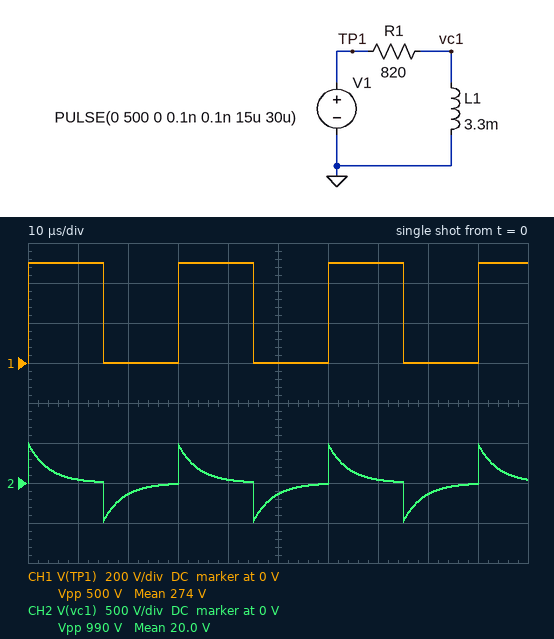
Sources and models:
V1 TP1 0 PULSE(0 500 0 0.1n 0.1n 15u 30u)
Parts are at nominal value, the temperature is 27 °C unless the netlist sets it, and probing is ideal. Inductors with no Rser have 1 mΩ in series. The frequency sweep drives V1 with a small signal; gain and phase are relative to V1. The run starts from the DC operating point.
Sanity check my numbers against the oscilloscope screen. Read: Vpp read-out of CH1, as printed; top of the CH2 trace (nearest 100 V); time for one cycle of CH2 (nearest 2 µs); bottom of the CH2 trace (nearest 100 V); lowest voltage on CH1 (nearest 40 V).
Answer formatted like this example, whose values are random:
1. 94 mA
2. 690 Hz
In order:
1. 500 V
2. 500 V
3. 30 µs
4. -500 V
5. 0 V
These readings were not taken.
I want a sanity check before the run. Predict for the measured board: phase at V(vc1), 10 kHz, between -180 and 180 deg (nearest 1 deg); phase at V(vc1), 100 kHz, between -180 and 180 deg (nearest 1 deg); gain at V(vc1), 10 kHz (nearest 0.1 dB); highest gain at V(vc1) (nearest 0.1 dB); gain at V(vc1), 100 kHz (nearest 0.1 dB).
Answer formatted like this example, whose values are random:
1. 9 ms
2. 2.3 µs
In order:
1. 76 deg
2. 22 deg
3. -12.2 dB
4. 0 dB
5. -0.6 dB
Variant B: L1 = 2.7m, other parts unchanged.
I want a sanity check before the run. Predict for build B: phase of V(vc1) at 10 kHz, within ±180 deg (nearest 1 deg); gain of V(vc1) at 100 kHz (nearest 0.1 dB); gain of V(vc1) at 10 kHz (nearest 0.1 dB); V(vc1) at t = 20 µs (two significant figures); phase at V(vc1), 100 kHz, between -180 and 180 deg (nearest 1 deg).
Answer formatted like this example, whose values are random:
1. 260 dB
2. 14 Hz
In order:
1. 78 deg
2. -0.9 dB
3. -13.9 dB
4. -110 V
5. 26 deg
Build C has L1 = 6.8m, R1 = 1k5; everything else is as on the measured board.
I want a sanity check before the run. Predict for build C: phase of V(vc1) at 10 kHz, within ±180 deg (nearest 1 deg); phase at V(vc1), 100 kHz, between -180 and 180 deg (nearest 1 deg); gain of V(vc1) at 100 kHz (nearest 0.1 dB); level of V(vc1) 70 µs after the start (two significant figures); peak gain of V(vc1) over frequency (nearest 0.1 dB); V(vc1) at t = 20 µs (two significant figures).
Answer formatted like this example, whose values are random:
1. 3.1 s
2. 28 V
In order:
1. 74 deg
2. 19 deg
3. -0.5 dB
4. 53 V
5. 0 dB
6. -160 V
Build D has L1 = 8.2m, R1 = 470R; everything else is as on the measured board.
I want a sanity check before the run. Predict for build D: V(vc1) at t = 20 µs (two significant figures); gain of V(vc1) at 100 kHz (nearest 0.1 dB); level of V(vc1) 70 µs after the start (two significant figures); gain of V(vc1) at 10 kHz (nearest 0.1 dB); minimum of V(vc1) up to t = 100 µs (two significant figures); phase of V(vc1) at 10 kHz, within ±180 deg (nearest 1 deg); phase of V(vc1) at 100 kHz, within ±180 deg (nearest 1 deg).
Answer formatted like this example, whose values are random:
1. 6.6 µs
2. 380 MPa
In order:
1. -220 V
2. 0 dB
3. 200 V
4. -2.6 dB
5. -350 V
6. 42 deg
7. 5 deg
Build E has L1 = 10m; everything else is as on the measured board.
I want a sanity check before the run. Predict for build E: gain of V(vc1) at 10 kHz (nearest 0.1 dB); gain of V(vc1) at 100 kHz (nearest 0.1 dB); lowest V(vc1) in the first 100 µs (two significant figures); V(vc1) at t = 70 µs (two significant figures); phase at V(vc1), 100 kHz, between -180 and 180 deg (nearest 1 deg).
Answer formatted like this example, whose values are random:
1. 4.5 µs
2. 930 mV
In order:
1. -4.3 dB
2. -0.1 dB
3. -390 V
4. 170 V
5. 7 deg
